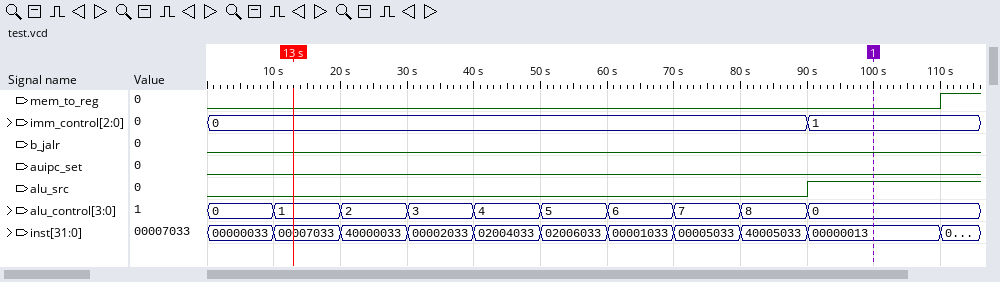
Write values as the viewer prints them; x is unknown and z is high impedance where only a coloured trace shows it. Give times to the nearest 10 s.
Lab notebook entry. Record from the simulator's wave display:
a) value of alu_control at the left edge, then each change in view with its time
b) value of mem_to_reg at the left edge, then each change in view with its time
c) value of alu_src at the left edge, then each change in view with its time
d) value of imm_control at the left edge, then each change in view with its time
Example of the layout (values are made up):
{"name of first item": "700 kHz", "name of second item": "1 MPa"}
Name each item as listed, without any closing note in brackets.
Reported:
{"value of alu_control at the left edge, then each change in view with its time": "0, 1 at 10 s, 2 at 20 s, 3 at 30 s, 4 at 40 s, 5 at 50 s, 6 at 60 s, 7 at 70 s, 8 at 80 s, 0 at 90 s", "value of mem_to_reg at the left edge, then each change in view with its time": "0, 1 at 110 s", "value of alu_src at the left edge, then each change in view with its time": "0, 1 at 90 s", "value of imm_control at the left edge, then each change in view with its time": "0, 1 at 90 s"}
